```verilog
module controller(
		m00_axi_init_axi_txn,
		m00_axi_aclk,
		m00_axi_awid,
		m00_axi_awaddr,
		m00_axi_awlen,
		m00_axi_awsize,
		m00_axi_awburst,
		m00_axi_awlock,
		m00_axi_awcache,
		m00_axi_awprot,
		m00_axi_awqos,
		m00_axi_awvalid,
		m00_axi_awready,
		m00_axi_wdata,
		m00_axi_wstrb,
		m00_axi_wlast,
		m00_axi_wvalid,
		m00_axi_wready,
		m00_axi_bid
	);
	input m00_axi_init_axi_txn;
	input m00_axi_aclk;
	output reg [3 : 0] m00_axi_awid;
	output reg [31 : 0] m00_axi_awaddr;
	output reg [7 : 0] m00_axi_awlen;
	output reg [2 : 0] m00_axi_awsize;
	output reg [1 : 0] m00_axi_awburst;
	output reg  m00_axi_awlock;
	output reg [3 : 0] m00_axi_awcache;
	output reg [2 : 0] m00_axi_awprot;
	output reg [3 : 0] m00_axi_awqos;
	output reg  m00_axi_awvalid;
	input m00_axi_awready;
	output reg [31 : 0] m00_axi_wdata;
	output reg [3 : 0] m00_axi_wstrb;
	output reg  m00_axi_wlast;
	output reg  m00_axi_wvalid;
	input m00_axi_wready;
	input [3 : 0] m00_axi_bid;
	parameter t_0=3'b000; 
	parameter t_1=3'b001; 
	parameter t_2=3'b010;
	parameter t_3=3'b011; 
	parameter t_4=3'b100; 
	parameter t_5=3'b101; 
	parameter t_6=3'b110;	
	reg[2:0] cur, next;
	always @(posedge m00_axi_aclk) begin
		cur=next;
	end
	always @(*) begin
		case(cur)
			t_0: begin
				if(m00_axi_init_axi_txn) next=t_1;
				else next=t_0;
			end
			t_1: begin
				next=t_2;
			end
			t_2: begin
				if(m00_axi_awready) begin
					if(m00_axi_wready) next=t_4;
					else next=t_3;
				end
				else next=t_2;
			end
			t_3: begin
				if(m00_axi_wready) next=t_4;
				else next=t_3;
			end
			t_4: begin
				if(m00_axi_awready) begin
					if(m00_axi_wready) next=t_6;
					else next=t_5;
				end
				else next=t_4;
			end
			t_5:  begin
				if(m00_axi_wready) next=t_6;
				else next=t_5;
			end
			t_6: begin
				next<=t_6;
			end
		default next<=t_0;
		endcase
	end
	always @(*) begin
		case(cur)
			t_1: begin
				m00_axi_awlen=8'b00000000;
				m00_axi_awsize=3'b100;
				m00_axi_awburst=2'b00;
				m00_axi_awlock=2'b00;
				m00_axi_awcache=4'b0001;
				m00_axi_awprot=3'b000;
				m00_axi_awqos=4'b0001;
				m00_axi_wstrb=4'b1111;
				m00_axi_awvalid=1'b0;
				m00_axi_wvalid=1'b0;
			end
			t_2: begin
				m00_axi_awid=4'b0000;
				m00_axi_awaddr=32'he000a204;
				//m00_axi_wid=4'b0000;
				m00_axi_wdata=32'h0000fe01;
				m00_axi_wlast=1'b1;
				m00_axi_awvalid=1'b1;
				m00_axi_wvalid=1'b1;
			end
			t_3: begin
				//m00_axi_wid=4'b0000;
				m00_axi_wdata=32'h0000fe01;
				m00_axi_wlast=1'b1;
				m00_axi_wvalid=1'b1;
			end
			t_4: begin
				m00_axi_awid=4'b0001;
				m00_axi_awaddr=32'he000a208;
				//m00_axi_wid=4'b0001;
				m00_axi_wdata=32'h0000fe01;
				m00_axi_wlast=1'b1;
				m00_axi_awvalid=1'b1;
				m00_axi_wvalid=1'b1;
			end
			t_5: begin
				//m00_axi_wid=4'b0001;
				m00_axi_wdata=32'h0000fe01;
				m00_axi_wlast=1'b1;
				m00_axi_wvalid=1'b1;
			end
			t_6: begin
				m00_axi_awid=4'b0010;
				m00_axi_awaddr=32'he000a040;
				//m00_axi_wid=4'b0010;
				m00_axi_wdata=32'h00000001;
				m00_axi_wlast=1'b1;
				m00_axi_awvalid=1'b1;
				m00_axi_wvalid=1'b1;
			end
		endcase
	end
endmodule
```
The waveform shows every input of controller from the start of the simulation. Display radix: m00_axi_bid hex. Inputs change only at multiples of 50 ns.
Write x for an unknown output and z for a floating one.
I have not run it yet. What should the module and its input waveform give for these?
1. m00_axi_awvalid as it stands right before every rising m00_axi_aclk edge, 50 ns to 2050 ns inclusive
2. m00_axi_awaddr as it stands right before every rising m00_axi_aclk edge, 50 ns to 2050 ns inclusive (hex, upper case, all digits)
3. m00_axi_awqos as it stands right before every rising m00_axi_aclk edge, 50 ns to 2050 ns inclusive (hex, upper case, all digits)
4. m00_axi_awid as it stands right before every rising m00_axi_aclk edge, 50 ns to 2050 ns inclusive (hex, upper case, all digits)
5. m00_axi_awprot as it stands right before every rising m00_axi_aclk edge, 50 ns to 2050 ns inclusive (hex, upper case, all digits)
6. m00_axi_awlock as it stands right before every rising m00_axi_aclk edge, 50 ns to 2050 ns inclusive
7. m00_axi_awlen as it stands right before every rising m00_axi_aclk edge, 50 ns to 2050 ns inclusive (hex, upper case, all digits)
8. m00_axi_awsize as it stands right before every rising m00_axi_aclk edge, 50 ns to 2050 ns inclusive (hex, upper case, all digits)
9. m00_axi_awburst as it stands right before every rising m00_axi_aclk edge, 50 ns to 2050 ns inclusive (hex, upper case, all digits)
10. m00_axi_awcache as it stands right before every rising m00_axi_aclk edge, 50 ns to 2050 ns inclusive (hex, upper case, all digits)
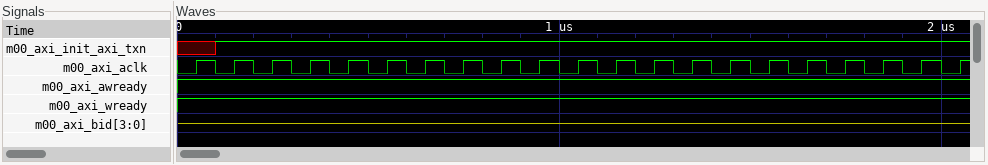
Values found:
x x 0 1 1 1 1 1 1 1 1 1 1 1 1 1 1 1 1 1 1
x, x, x, E000A204, E000A208, E000A040, E000A040, E000A040, E000A040, E000A040, E000A040, E000A040, E000A040, E000A040, E000A040, E000A040, E000A040, E000A040, E000A040, E000A040, E000A040
x, x, 1, 1, 1, 1, 1, 1, 1, 1, 1, 1, 1, 1, 1, 1, 1, 1, 1, 1, 1
x, x, x, 0, 1, 2, 2, 2, 2, 2, 2, 2, 2, 2, 2, 2, 2, 2, 2, 2, 2
x, x, 0, 0, 0, 0, 0, 0, 0, 0, 0, 0, 0, 0, 0, 0, 0, 0, 0, 0, 0
x x 0 0 0 0 0 0 0 0 0 0 0 0 0 0 0 0 0 0 0
x, x, 00, 00, 00, 00, 00, 00, 00, 00, 00, 00, 00, 00, 00, 00, 00, 00, 00, 00, 00
x, x, 4, 4, 4, 4, 4, 4, 4, 4, 4, 4, 4, 4, 4, 4, 4, 4, 4, 4, 4
x, x, 0, 0, 0, 0, 0, 0, 0, 0, 0, 0, 0, 0, 0, 0, 0, 0, 0, 0, 0
x, x, 1, 1, 1, 1, 1, 1, 1, 1, 1, 1, 1, 1, 1, 1, 1, 1, 1, 1, 1
